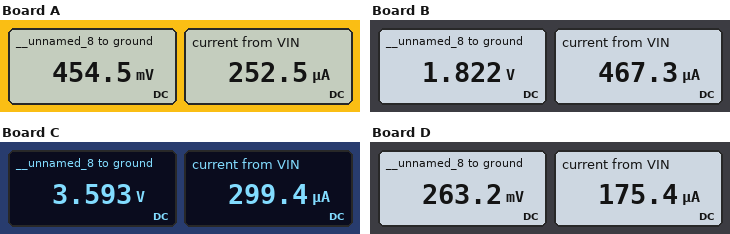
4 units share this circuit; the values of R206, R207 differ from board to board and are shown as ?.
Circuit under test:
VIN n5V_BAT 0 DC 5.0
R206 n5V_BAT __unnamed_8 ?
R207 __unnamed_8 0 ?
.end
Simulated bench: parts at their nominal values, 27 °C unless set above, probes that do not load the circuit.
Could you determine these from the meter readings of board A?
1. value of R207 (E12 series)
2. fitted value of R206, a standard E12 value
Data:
1.8 kΩ
18 kΩ
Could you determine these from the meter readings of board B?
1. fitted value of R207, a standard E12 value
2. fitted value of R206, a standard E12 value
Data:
3.9 kΩ
6.8 kΩ
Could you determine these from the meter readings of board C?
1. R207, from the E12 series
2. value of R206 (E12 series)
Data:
12 kΩ
4.7 kΩ
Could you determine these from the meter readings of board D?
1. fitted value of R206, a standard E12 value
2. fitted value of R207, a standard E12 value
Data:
27 kΩ
1.5 kΩ
